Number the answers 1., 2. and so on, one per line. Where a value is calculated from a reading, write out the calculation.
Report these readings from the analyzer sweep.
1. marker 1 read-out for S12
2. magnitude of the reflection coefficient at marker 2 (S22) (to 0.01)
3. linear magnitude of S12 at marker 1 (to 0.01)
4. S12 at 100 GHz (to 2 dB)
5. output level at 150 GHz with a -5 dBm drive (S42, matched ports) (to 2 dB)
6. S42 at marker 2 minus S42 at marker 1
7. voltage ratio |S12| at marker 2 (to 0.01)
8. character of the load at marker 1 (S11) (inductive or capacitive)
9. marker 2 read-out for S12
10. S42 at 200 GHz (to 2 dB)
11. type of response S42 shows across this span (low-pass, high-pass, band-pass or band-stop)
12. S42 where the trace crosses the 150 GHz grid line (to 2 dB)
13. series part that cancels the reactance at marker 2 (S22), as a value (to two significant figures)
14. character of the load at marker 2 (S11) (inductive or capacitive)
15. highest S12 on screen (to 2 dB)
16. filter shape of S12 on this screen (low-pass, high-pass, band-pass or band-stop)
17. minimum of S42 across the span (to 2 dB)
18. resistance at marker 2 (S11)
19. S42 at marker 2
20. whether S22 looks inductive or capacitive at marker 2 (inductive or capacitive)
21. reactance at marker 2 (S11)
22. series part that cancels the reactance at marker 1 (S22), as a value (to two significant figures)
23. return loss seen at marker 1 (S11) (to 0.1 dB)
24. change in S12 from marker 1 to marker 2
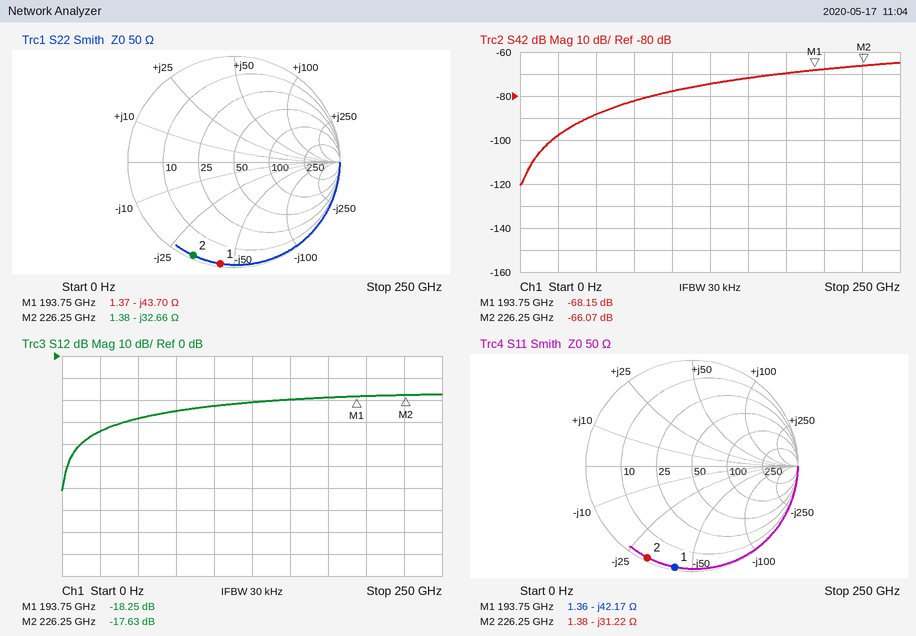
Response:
1. -18.25 dB
2. 0.96
3. 10^(-18.25/20) ≈ 0.12
4. -22 dB
5. -5 dBm + (-72 dB) = -76 dBm
6. -66.07 − (-68.15) = 2.08 dB
7. 10^(-17.63/20) ≈ 0.13
8. capacitive
9. -17.63 dB
10. -68 dB
11. high-pass
12. -72 dB
13. L = 32.66 Ω/(2π × 226.25 GHz) ≈ 23 pH
14. capacitive
15. -18 dB
16. high-pass
17. -120 dB
18. 1.38 Ω
19. -66.07 dB
20. capacitive
21. -31.22 Ω
22. L = 43.7 Ω/(2π × 193.75 GHz) ≈ 36 pH
23. 0.3 dB
24. -17.63 − (-18.25) = 0.62 dB
